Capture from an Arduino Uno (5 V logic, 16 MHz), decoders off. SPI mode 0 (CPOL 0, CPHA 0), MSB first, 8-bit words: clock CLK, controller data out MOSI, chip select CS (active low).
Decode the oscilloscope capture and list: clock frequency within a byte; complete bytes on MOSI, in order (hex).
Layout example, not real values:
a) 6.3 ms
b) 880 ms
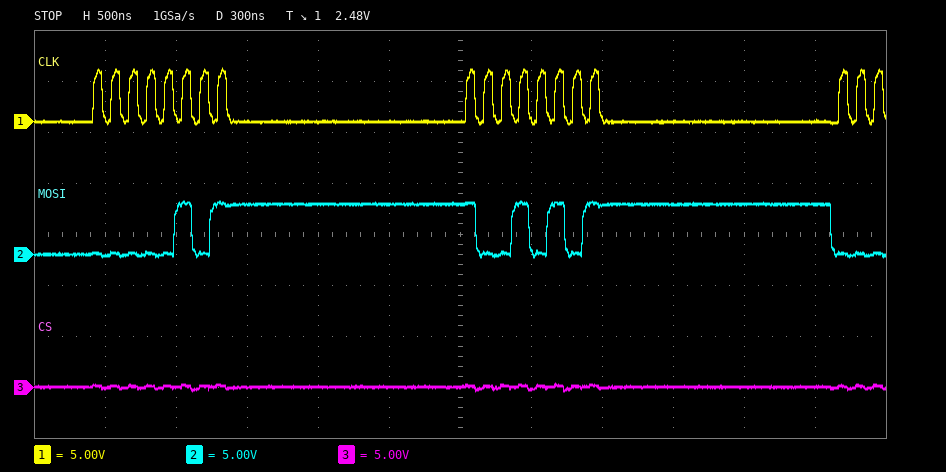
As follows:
a) 8 MHz
b) 05 95
